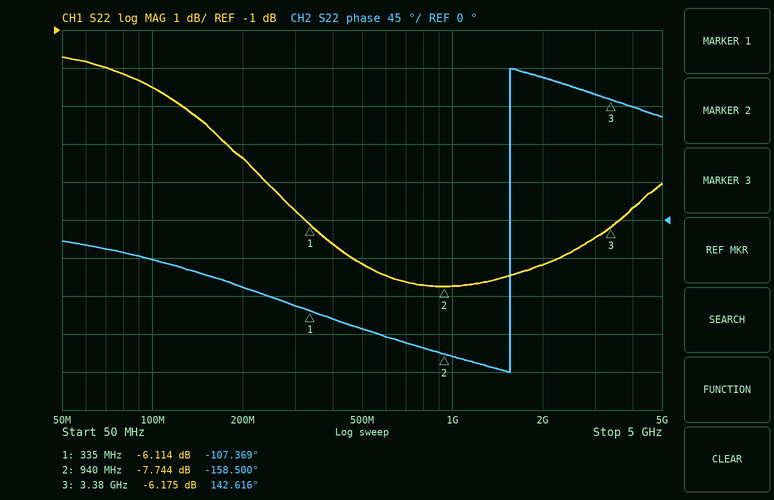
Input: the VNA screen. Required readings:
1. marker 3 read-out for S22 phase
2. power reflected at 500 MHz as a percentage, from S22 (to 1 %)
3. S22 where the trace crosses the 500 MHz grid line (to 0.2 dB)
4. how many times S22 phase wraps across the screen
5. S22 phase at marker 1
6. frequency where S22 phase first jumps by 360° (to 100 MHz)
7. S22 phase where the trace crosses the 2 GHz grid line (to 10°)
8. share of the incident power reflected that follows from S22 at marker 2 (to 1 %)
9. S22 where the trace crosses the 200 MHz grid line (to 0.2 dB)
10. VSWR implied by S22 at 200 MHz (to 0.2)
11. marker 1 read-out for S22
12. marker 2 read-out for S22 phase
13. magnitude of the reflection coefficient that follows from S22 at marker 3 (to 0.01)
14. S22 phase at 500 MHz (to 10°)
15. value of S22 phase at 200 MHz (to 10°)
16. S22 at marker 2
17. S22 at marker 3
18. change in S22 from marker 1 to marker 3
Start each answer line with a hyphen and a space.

- 142.616°
- 19 %
- -7.2 dB
- 1
- -107.369°
- 1.6 GHz
- 170°
- 17 %
- -4.4 dB
- 4.0
- -6.114 dB
- -158.500°
- 0.49
- -130°
- -80°
- -7.744 dB
- -6.175 dB
- -0.061 dB
